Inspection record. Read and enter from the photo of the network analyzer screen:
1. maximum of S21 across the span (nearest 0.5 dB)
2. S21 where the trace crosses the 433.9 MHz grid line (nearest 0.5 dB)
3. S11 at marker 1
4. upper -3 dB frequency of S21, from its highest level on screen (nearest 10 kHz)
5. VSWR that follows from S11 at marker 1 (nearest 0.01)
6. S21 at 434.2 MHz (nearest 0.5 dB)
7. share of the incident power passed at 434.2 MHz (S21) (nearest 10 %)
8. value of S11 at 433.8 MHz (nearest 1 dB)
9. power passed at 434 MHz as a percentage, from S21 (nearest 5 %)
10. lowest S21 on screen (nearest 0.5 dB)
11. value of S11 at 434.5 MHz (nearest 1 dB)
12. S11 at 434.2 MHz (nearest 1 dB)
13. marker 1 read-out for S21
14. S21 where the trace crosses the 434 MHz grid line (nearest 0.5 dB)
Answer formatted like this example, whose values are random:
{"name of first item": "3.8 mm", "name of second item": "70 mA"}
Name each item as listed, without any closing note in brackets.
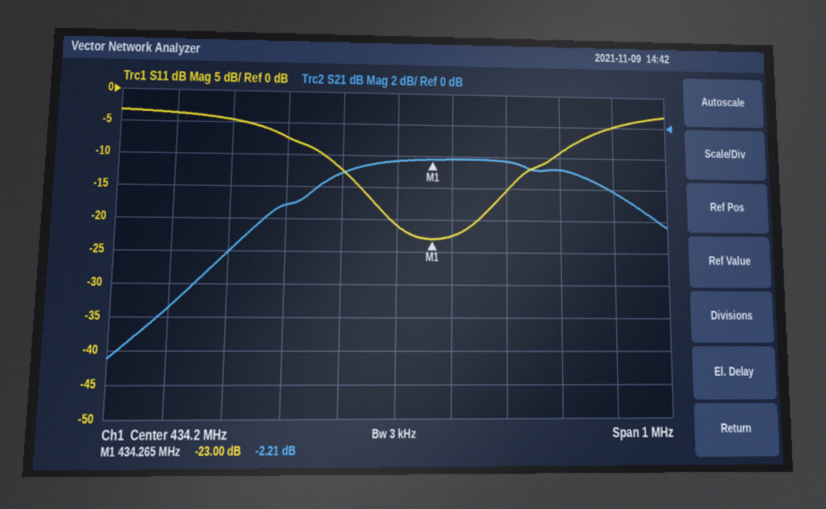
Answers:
{"maximum of S21 across the span": "-2.0 dB", "S21 where the trace crosses the 433.9 MHz grid line": "-8.0 dB", "S11 at marker 1": "-23.00 dB", "upper -3 dB frequency of S21, from its highest level on screen": "434.65 MHz", "VSWR that follows from S11 at marker 1": "1.15", "S21 at 434.2 MHz": "-2.5 dB", "share of the incident power passed at 434.2 MHz (S21)": "60 %", "value of S11 at 433.8 MHz": "-4 dB", "power passed at 434 MHz as a percentage, from S21": "30 %", "lowest S21 on screen": "-14.5 dB", "value of S11 at 434.5 MHz": "-9 dB", "S11 at 434.2 MHz": "-21 dB", "marker 1 read-out for S21": "-2.21 dB", "S21 where the trace crosses the 434 MHz grid line": "-5.0 dB"}
